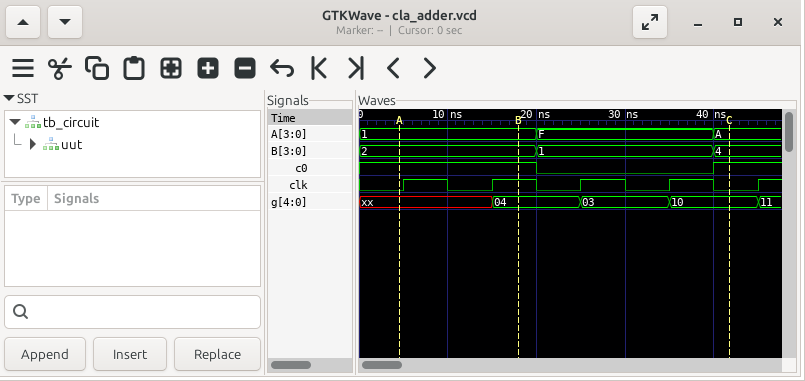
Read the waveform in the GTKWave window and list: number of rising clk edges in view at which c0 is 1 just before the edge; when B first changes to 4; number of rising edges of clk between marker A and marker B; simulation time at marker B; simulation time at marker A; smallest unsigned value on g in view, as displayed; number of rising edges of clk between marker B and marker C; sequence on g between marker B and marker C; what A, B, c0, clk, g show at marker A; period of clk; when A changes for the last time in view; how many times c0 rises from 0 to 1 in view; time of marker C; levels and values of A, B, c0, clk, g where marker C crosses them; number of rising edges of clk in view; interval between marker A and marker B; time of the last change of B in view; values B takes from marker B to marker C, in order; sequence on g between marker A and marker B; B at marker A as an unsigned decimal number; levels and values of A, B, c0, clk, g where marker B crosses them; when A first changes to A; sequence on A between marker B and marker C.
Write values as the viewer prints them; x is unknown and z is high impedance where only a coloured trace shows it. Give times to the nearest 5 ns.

3
40 ns
2
20 ns
5 ns
03
2
04, 03, 10
A=1, B=2, c0=1, clk=0, g=xx
10 ns
40 ns
1
40 ns
A=A, B=4, c0=1, clk=0, g=10
5
15 ns
40 ns
2, 1, 4
xx, 04
2
A=1, B=2, c0=1, clk=1, g=04
40 ns
1, F, A
